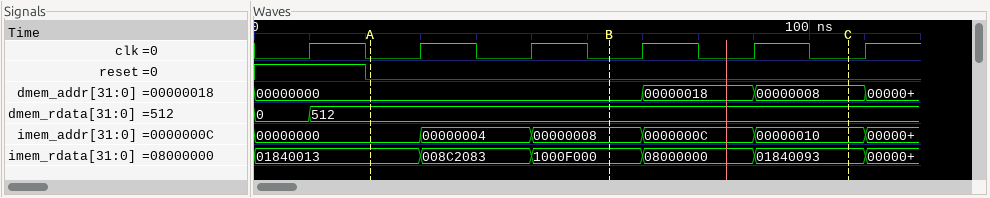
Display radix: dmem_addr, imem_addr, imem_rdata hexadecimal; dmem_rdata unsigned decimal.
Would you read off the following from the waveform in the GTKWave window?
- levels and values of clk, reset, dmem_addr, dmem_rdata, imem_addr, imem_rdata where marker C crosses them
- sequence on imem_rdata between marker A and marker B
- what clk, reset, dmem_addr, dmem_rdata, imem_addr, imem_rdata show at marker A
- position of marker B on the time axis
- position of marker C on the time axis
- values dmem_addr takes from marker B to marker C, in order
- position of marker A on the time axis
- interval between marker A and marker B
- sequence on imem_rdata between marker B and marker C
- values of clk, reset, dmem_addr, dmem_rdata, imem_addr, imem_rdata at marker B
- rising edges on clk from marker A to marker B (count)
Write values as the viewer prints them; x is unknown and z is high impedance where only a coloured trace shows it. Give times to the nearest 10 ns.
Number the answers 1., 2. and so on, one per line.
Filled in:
1. clk=0, reset=0, dmem_addr=00000008, dmem_rdata=512, imem_addr=00000010, imem_rdata=01840093
2. 01840013, 008C2083, 1000F000
3. clk=0, reset=0, dmem_addr=00000000, dmem_rdata=512, imem_addr=00000000, imem_rdata=01840013
4. 60 ns
5. 110 ns
6. 00000000, 00000018, 00000008
7. 20 ns
8. 40 ns
9. 1000F000, 08000000, 01840093
10. clk=0, reset=0, dmem_addr=00000000, dmem_rdata=512, imem_addr=00000008, imem_rdata=1000F000
11. 2
